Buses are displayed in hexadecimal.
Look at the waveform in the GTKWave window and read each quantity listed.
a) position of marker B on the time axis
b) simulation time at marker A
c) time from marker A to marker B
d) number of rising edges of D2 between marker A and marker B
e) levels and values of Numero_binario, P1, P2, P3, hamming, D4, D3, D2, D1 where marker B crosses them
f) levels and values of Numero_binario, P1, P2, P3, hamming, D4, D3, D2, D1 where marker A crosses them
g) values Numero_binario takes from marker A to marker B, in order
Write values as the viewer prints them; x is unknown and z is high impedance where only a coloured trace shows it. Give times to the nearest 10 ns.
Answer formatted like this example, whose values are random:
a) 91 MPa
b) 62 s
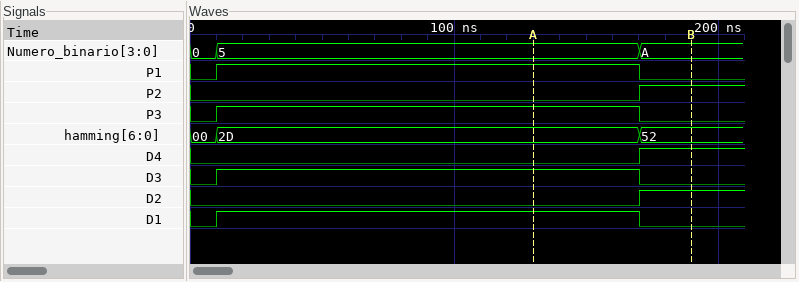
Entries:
a) 190 ns
b) 130 ns
c) 60 ns
d) 1
e) Numero_binario=A, P1=0, P2=1, P3=0, hamming=52, D4=1, D3=0, D2=1, D1=0
f) Numero_binario=5, P1=1, P2=0, P3=1, hamming=2D, D4=0, D3=1, D2=0, D1=1
g) 5, A
